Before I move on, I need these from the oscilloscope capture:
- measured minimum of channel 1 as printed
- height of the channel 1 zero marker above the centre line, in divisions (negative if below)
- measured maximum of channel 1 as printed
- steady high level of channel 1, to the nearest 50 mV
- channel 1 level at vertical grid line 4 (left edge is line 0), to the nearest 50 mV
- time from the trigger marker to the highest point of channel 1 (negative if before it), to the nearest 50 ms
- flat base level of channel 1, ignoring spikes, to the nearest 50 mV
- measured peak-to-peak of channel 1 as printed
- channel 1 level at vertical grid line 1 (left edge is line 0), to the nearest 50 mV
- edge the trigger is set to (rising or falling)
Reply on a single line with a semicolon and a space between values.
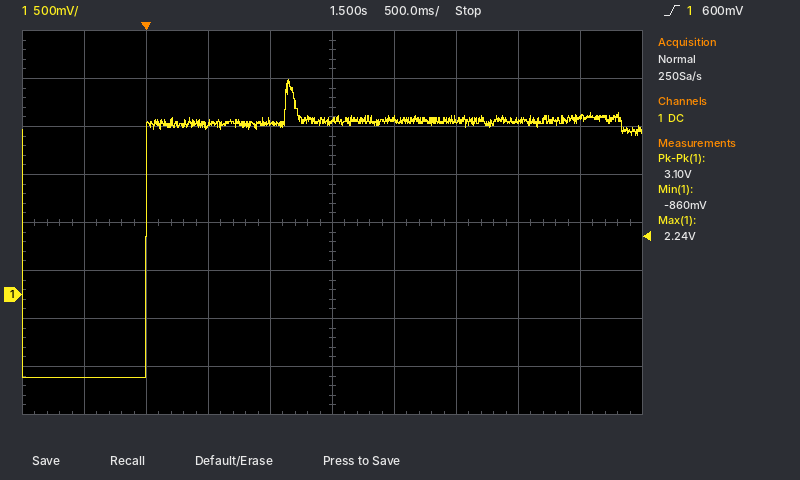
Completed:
-860 mV; -1.5 div; 2.24 V; 1.80 V; 1.80 V; +1.15 s; -850 mV; 3.10 V; -850 mV; rising
